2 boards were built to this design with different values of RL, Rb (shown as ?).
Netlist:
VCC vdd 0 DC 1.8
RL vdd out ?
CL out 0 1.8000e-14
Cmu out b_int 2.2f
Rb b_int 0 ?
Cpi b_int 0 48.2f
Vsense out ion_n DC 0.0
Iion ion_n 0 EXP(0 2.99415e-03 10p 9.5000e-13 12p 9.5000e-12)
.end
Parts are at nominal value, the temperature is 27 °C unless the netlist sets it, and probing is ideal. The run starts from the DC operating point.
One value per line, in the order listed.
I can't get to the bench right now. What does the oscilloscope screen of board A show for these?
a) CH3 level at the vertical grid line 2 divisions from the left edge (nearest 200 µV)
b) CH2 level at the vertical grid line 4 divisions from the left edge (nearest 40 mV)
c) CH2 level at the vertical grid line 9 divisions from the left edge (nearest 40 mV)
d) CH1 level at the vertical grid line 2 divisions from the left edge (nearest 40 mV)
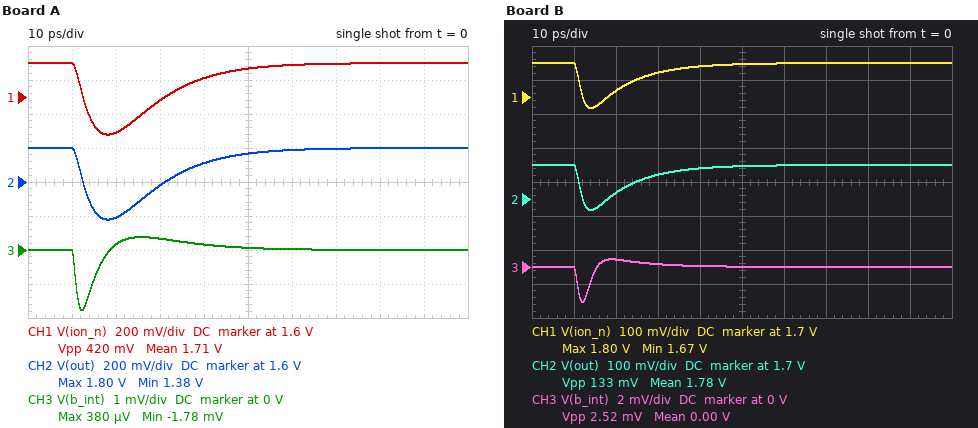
200 µV
1.72 V
1.80 V
1.40 V
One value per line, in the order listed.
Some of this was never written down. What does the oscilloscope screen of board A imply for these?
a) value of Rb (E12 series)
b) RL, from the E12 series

8.2 Ω
270 Ω
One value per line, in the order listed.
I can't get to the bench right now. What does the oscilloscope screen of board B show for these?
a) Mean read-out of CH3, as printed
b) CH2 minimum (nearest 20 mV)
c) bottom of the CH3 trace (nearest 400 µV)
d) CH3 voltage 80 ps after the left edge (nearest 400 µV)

0.00 V
1.66 V
-2.0 mV
0 V
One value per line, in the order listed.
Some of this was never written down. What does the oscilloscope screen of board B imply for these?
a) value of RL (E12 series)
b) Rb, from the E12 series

56 Ω
22 Ω
